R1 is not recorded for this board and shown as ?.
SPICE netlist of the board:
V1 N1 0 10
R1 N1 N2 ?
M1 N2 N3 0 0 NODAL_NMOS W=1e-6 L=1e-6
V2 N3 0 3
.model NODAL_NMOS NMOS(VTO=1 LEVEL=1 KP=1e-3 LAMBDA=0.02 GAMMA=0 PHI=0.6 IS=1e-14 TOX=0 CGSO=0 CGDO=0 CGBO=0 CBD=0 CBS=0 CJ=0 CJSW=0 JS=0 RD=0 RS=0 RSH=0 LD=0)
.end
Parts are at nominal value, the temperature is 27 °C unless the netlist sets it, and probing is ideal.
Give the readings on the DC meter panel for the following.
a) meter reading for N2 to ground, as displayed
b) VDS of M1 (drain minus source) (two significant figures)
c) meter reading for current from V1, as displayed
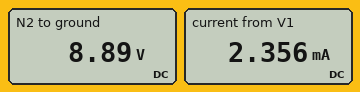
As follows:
8.89 V
8.9 V
2.356 mA
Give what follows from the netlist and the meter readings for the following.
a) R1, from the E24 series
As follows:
470 Ω
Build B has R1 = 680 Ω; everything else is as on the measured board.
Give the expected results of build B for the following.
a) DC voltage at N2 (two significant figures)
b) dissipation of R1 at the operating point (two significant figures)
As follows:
8.4 V
3.7 mW
